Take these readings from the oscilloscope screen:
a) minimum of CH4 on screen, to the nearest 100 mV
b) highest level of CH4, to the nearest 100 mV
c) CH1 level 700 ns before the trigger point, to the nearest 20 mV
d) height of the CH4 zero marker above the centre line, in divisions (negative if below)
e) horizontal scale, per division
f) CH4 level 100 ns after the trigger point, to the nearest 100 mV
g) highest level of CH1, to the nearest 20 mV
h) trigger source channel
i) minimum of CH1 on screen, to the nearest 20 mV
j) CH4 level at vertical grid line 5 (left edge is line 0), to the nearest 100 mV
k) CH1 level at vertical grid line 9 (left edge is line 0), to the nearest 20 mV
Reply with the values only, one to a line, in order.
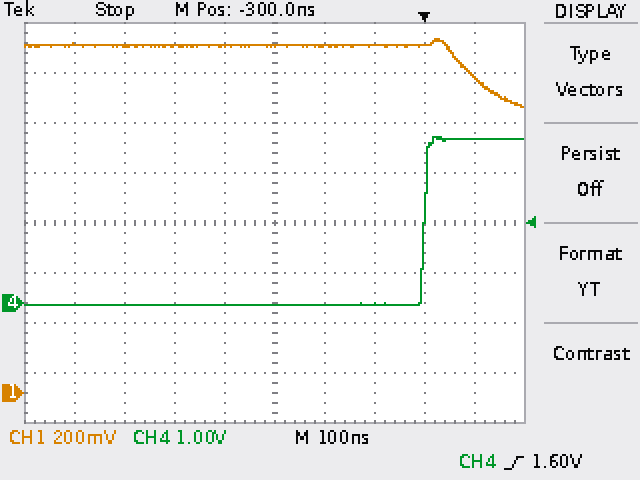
0.0 V
3.3 V
1.40 V
-1.6 div
100 ns
3.3 V
1.42 V
CH4
1.14 V
0.0 V
1.26 V
